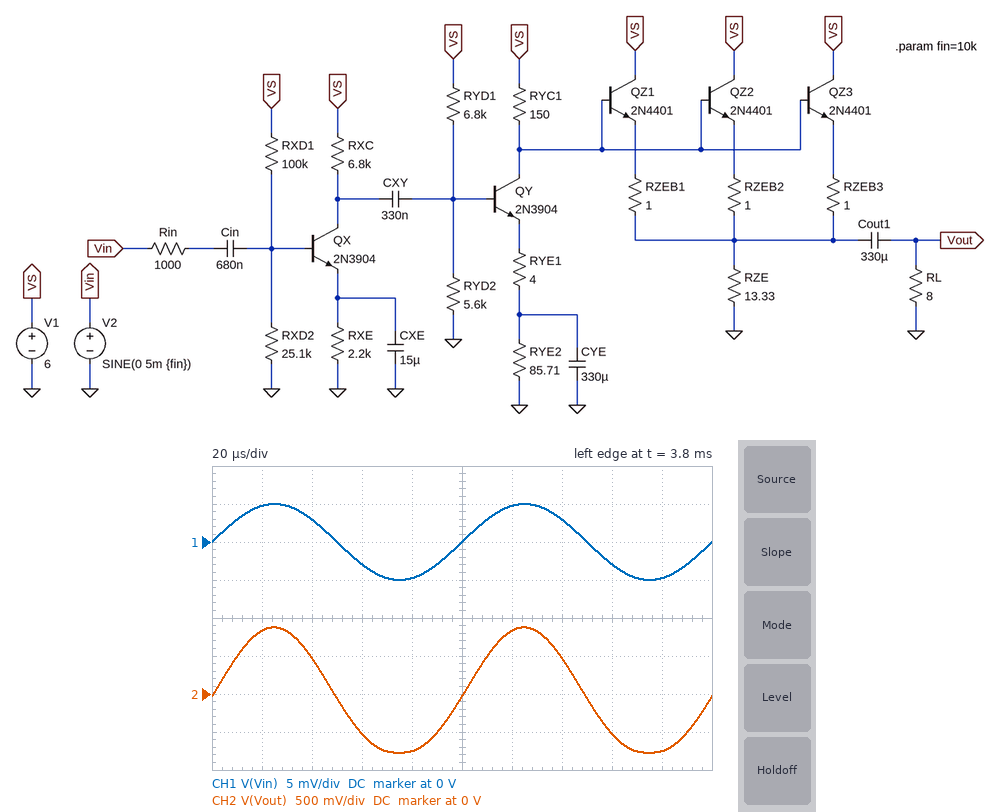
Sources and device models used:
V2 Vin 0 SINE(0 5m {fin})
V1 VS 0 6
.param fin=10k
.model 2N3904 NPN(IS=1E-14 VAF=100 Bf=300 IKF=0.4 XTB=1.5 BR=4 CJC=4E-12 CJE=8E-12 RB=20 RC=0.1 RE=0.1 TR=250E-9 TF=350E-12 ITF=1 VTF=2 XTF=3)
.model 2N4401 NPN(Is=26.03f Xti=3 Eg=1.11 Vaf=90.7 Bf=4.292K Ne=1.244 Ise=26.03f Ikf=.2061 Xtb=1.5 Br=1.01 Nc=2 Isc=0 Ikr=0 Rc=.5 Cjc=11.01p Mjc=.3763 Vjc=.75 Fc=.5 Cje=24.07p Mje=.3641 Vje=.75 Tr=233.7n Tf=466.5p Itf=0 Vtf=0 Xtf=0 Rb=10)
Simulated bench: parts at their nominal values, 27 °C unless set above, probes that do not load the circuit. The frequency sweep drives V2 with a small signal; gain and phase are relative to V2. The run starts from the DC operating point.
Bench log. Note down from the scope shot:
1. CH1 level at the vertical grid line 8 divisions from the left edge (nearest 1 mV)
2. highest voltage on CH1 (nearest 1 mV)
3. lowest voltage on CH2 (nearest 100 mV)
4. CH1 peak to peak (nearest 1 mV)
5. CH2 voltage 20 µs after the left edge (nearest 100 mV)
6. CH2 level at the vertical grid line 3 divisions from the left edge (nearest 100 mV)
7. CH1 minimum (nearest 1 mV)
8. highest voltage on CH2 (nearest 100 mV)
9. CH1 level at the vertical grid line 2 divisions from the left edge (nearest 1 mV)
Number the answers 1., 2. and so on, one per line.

1. -3 mV
2. 5 mV
3. -800 mV
4. 10 mV
5. 800 mV
6. -500 mV
7. -5 mV
8. 900 mV
9. 3 mV
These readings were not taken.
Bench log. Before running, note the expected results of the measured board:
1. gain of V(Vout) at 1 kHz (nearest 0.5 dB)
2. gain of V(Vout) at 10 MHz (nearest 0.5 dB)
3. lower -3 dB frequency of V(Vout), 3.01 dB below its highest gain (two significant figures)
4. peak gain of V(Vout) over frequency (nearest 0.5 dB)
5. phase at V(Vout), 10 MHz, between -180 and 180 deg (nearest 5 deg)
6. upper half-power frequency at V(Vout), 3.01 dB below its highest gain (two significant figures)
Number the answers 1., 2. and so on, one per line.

1. 44.5 dB
2. 20.5 dB
3. 170 Hz
4. 44.5 dB
5. -155 deg
6. 960 kHz
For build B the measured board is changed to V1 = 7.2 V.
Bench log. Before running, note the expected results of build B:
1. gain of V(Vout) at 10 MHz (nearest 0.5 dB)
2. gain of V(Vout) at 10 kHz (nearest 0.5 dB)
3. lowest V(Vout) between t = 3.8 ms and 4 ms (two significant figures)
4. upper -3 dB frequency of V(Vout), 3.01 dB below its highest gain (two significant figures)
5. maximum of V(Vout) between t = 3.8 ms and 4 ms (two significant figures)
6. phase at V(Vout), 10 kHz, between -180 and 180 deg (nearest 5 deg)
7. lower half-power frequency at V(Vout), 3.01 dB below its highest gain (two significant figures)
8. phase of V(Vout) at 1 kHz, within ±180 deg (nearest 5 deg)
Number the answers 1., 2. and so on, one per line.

1. 23.0 dB
2. 47.5 dB
3. -840 mV
4. 920 kHz
5. 1.2 V
6. 0 deg
7. 200 Hz
8. 20 deg
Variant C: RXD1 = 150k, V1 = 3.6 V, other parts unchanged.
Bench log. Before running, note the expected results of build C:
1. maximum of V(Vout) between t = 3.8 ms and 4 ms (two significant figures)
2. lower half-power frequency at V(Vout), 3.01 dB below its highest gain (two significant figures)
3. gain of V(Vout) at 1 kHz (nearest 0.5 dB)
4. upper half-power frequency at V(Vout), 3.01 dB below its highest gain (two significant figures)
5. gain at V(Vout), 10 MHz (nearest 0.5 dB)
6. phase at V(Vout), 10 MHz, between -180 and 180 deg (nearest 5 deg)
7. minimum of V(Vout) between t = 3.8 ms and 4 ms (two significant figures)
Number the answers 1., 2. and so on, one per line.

1. 12 mV
2. 100 Hz
3. 7.0 dB
4. 1.2 MHz
5. -11.5 dB
6. 165 deg
7. -11 mV
